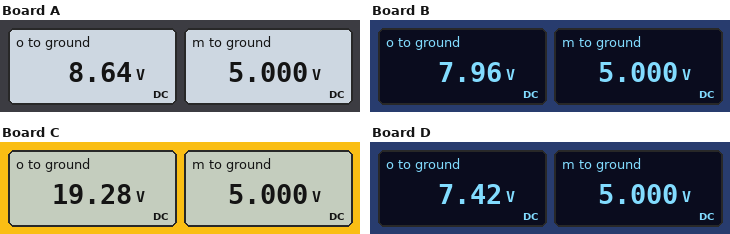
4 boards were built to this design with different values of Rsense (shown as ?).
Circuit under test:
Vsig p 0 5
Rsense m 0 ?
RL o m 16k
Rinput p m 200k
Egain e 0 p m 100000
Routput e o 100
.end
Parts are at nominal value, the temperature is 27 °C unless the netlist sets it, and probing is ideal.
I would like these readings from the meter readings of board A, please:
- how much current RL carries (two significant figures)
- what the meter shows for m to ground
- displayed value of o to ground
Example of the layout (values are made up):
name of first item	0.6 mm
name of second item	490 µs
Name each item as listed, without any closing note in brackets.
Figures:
how much current RL carries	230 µA
what the meter shows for m to ground	5.000 V
displayed value of o to ground	8.64 V
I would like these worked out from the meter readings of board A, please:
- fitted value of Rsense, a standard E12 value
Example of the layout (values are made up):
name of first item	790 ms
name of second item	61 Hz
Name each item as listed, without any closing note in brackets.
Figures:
fitted value of Rsense, a standard E12 value	22 kΩ
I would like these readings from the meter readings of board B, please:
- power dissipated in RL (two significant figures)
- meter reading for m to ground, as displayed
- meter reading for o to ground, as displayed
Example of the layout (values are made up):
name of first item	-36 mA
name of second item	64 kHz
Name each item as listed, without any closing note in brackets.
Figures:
power dissipated in RL	550 µW
meter reading for m to ground, as displayed	5.000 V
meter reading for o to ground, as displayed	7.96 V
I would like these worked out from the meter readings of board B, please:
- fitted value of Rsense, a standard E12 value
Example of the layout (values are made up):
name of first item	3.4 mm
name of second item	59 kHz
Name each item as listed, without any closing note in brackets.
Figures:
fitted value of Rsense, a standard E12 value	27 kΩ
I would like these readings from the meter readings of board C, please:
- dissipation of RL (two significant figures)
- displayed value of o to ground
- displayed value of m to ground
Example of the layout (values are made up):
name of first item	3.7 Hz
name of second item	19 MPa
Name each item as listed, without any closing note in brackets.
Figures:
dissipation of RL	13 mW
displayed value of o to ground	19.28 V
displayed value of m to ground	5.000 V
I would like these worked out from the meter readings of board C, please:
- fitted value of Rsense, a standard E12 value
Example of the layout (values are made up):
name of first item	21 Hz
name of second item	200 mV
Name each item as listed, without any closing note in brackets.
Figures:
fitted value of Rsense, a standard E12 value	5.6 kΩ
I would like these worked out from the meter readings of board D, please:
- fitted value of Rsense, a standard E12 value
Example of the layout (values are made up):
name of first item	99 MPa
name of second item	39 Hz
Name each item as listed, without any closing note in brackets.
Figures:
fitted value of Rsense, a standard E12 value	33 kΩ
